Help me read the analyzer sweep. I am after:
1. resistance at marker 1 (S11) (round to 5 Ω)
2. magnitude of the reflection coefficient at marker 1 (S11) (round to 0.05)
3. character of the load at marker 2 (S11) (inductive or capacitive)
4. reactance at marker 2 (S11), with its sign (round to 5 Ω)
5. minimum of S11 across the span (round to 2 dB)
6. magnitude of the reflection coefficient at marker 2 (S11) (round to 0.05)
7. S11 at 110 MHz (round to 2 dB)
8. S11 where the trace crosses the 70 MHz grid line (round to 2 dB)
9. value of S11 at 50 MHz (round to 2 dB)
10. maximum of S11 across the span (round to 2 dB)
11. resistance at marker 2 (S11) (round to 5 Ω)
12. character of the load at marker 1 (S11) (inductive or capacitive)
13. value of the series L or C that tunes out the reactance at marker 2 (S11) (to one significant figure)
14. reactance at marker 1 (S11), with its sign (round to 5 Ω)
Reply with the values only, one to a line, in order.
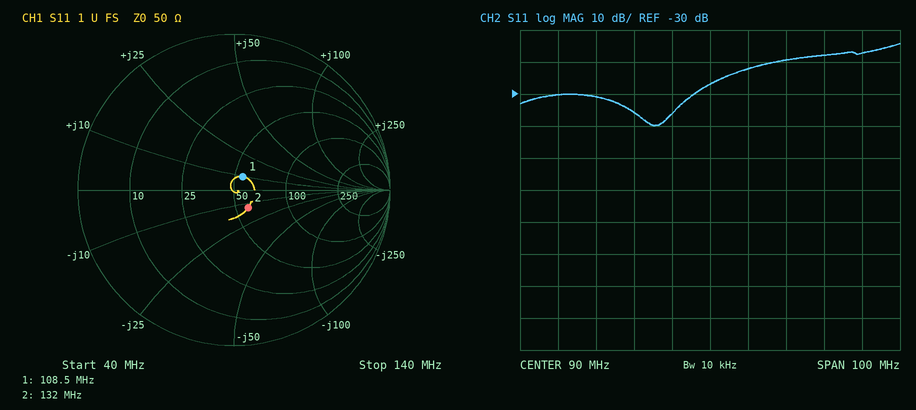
55 Ω
0.10
capacitive
-15 Ω
-40 dB
0.15
-20 dB
-36 dB
-30 dB
-14 dB
60 Ω
inductive
20 nH
+10 Ω
